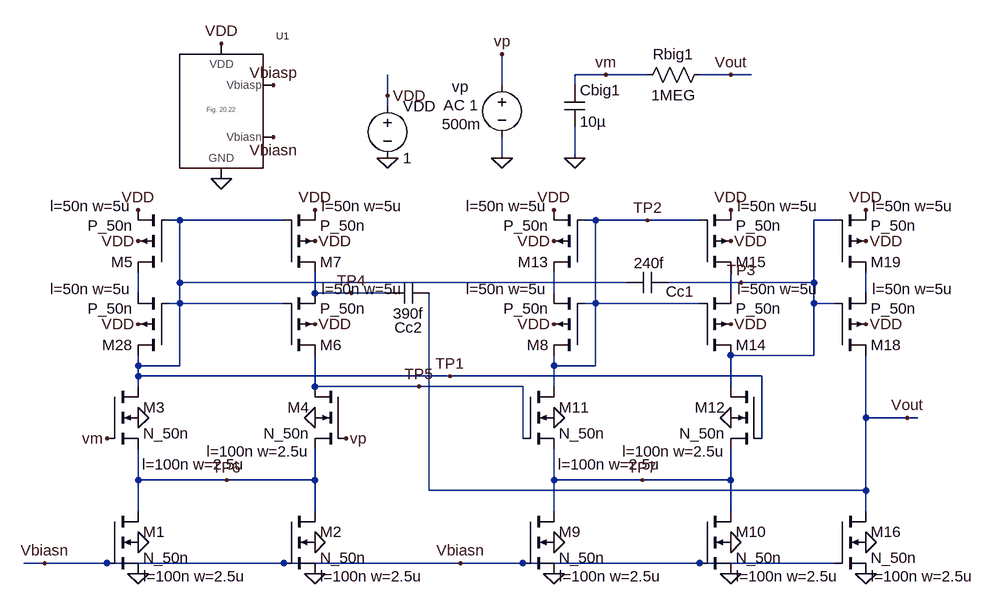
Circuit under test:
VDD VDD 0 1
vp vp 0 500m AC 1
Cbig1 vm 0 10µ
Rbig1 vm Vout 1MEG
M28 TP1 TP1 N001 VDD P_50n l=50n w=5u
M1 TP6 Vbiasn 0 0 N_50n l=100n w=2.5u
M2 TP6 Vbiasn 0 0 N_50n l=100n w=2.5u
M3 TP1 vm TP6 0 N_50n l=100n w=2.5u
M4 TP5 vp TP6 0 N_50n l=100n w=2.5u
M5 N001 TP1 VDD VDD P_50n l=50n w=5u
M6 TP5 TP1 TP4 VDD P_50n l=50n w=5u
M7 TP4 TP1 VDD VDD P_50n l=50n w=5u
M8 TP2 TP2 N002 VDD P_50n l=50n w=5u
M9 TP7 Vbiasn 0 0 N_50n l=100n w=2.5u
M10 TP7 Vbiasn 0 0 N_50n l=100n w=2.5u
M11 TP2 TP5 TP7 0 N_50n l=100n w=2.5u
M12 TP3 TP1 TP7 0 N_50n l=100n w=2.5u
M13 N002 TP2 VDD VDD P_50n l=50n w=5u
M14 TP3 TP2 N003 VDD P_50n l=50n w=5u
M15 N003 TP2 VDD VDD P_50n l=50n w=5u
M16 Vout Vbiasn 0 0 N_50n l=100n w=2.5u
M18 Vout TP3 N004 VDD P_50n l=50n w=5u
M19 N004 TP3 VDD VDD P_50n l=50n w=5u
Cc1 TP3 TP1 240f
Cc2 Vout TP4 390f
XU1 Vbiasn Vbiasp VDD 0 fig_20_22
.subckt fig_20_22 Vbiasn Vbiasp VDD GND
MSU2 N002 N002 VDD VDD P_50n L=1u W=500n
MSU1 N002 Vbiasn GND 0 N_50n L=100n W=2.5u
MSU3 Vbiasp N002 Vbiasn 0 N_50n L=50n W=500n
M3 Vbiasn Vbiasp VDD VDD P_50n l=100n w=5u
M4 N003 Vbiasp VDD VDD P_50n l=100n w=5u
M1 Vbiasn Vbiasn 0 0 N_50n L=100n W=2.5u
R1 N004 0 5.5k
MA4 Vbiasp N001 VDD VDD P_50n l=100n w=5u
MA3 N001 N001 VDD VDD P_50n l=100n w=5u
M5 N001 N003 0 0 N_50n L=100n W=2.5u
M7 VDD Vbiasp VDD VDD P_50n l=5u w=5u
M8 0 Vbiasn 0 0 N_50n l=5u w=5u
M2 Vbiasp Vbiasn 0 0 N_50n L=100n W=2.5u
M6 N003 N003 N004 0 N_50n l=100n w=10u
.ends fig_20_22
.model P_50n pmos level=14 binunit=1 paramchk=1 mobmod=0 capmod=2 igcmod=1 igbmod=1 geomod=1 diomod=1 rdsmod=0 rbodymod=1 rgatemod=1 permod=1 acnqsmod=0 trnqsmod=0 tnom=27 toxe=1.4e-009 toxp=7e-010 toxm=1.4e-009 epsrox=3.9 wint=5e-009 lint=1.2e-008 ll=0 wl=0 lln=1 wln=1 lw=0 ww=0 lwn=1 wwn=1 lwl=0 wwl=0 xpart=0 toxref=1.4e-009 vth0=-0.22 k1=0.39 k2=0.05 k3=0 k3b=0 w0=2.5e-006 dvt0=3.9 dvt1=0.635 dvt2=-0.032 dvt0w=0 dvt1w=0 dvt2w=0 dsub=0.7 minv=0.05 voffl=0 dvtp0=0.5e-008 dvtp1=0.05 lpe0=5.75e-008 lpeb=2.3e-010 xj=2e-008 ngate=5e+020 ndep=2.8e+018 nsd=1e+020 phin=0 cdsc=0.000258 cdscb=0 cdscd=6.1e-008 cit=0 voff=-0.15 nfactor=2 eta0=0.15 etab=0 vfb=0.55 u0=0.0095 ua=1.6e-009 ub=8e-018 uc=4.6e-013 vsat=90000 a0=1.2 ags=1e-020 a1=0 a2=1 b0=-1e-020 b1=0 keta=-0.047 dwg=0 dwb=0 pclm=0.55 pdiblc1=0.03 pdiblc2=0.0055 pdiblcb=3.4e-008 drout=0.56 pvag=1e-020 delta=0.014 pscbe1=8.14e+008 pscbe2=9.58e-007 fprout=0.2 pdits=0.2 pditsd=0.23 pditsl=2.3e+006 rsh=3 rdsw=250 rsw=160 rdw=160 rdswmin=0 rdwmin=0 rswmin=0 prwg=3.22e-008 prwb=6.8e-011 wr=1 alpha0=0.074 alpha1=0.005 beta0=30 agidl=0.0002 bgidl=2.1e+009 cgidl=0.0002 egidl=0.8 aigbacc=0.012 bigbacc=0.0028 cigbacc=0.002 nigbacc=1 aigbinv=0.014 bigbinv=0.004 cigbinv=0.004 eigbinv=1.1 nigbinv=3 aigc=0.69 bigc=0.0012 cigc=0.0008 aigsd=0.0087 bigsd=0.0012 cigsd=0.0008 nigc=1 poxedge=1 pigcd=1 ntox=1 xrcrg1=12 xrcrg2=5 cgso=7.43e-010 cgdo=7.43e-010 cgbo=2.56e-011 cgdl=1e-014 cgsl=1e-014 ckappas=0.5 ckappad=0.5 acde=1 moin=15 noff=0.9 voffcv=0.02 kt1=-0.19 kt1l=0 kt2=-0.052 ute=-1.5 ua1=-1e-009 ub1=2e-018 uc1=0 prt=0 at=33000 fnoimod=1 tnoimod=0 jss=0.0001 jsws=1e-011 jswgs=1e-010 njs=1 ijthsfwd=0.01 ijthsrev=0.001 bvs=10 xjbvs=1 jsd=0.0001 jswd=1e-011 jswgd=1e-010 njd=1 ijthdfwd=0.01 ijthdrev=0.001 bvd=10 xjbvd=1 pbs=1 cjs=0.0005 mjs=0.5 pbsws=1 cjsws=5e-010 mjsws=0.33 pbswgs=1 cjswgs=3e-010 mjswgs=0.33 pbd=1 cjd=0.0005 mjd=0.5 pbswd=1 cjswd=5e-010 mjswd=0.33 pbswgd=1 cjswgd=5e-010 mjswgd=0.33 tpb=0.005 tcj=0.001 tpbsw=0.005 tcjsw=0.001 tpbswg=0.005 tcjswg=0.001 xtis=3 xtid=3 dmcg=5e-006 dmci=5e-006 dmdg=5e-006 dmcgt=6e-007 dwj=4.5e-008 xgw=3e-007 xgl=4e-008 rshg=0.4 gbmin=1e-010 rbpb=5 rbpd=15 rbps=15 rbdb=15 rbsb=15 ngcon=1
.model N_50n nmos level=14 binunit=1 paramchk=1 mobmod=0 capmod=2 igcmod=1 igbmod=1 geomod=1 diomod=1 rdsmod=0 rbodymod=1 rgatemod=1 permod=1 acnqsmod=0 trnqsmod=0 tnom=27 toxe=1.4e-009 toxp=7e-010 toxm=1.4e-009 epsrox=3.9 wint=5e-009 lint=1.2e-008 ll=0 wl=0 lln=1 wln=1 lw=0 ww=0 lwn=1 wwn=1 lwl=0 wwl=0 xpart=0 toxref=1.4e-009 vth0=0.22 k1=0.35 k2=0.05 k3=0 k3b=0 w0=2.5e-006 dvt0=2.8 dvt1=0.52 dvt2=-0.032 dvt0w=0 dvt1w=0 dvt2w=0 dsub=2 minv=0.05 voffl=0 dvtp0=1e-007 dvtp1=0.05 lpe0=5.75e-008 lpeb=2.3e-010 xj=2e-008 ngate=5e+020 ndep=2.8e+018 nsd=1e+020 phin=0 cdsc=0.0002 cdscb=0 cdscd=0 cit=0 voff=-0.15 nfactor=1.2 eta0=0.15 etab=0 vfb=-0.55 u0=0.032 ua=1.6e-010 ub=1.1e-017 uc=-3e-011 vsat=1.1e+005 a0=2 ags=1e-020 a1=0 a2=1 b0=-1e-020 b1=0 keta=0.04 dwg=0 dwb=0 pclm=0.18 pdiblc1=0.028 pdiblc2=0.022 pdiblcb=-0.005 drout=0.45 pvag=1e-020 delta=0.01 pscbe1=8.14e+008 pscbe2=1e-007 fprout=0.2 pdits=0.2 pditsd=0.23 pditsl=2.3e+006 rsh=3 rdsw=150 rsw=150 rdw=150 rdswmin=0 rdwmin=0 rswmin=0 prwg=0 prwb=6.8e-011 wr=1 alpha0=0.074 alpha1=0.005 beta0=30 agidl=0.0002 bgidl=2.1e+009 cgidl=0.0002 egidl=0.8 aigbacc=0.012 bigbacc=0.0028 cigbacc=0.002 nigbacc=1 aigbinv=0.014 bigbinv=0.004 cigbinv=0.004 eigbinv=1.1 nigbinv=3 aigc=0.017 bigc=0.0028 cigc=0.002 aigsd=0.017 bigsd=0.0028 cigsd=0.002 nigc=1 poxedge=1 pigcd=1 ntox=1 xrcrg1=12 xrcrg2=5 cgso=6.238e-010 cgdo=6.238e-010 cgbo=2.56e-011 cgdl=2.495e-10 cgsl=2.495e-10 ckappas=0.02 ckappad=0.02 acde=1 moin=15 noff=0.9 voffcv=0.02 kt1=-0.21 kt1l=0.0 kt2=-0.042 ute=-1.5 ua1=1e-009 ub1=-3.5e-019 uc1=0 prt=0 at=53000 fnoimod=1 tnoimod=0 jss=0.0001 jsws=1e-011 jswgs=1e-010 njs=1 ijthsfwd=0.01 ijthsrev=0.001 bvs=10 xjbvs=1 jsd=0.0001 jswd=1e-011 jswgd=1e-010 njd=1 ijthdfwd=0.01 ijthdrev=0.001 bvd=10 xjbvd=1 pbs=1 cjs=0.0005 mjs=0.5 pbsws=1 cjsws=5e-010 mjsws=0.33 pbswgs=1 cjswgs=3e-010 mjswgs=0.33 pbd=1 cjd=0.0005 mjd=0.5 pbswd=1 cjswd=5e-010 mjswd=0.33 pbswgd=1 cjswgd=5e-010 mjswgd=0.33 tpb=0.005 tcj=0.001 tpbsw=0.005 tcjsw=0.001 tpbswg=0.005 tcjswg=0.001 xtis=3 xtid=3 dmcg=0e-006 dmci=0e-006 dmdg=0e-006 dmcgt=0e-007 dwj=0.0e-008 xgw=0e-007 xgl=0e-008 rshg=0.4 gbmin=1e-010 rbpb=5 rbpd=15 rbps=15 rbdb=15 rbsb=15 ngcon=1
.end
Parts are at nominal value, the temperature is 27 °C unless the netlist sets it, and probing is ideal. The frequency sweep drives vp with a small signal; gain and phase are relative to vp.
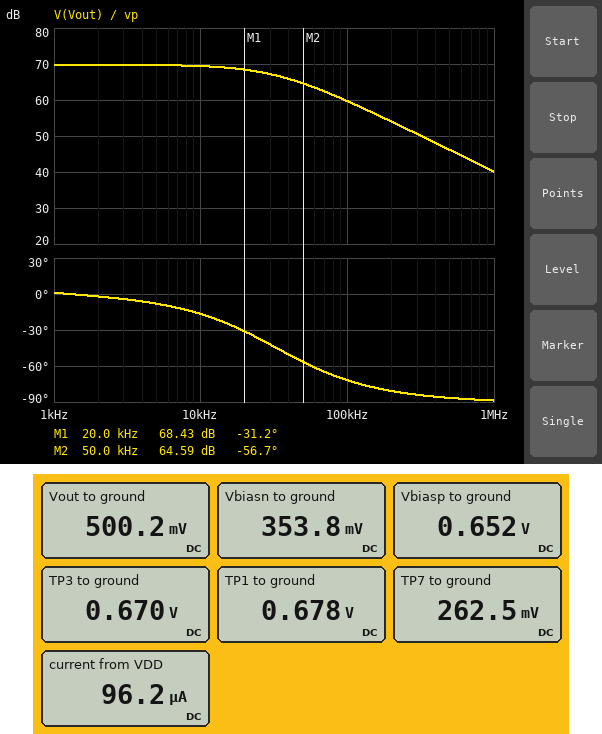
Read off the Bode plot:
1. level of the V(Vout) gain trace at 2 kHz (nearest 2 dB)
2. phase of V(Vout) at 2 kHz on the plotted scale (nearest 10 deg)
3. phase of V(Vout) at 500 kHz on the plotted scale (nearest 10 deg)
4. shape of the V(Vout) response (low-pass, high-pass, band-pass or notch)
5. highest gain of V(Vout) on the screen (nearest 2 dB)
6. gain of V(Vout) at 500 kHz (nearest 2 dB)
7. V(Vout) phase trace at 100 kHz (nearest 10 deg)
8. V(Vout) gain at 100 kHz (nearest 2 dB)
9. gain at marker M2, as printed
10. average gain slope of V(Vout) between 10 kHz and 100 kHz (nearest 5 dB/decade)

70 dB
0 deg
-90 deg
low-pass
70 dB
46 dB
-70 deg
60 dB
64.59 dB
-10 dB/decade
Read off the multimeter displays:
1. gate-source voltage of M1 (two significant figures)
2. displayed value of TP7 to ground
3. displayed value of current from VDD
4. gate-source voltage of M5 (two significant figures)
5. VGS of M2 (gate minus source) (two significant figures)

350 mV
262.5 mV
96.2 µA
-320 mV
350 mV
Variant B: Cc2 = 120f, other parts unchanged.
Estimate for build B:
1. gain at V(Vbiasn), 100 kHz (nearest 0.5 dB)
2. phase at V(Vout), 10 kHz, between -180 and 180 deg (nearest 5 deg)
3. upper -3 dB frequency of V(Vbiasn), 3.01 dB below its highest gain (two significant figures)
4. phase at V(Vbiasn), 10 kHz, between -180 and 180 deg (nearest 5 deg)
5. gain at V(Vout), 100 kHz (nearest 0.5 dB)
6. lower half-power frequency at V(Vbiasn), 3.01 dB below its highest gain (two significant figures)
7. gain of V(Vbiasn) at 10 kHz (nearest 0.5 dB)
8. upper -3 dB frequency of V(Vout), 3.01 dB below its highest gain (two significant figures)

-31.0 dB
-5 deg
15 MHz
45 deg
66.5 dB
90 kHz
-45.5 dB
92 kHz
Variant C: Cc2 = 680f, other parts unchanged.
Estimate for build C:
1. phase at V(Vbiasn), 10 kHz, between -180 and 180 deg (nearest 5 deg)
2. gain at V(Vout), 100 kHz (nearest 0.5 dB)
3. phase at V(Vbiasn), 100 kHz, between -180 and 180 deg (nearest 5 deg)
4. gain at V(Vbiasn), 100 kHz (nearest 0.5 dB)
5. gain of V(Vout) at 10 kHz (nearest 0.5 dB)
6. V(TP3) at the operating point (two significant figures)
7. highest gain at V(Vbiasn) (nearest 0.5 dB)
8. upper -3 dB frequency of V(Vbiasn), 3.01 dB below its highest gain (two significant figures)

25 deg
55.5 dB
5 deg
-42.0 dB
69.0 dB
670 mV
-41.5 dB
24 MHz
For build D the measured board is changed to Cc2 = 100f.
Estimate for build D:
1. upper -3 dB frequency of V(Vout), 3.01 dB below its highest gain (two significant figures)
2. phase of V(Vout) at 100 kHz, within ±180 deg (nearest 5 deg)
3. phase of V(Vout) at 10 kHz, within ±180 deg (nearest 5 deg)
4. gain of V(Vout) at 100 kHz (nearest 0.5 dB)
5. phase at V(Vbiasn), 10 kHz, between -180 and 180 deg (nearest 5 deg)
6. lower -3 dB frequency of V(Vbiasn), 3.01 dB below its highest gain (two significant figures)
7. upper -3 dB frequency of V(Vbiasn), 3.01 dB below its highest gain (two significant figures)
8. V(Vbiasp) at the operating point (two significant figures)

110 kHz
-45 deg
-5 deg
67.0 dB
45 deg
100 kHz
15 MHz
650 mV
